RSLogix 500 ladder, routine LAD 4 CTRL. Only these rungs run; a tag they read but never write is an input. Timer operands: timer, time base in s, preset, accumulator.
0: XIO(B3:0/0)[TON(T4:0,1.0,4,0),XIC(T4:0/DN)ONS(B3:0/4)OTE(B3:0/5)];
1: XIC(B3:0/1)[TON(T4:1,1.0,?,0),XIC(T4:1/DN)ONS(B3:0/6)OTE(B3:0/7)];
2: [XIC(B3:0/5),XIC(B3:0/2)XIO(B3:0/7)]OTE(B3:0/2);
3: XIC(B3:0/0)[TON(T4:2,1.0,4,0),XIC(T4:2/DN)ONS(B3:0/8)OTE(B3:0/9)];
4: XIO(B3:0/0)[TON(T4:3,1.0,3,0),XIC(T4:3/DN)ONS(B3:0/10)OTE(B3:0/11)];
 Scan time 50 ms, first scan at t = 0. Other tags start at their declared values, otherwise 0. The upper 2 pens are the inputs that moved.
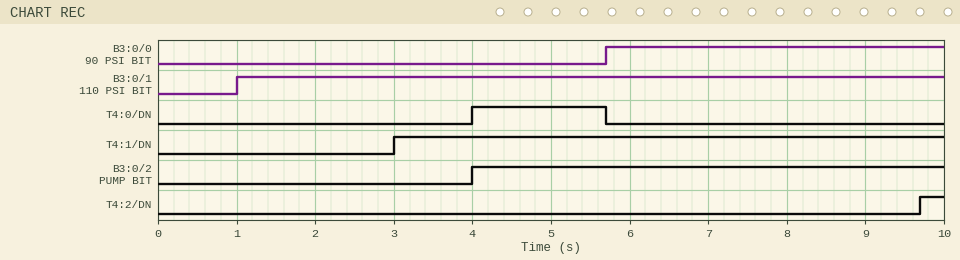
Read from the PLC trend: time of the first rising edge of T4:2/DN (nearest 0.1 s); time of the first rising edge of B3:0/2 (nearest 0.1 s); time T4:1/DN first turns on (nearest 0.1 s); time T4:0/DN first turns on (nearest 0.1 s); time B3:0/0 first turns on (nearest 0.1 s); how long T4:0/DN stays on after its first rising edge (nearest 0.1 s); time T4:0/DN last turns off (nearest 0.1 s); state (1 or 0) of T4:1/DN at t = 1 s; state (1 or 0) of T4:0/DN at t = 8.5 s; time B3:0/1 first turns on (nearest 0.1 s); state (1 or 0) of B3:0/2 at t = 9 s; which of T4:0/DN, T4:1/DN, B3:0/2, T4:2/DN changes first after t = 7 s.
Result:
9.7 s
4.0 s
3.0 s
4.0 s
5.7 s
1.7 s
5.7 s
0
0
1.0 s
1
T4:2/DN
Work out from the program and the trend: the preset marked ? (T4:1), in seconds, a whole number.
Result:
2 s
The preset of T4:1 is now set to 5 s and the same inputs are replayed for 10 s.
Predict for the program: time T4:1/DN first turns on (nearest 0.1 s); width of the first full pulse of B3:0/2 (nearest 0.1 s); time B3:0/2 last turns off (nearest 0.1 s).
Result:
6.0 s
2.0 s
6.0 s
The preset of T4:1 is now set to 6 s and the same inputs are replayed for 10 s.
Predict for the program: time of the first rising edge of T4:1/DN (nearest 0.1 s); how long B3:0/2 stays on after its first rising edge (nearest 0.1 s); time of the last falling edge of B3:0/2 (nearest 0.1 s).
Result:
7.0 s
3.0 s
7.0 s
